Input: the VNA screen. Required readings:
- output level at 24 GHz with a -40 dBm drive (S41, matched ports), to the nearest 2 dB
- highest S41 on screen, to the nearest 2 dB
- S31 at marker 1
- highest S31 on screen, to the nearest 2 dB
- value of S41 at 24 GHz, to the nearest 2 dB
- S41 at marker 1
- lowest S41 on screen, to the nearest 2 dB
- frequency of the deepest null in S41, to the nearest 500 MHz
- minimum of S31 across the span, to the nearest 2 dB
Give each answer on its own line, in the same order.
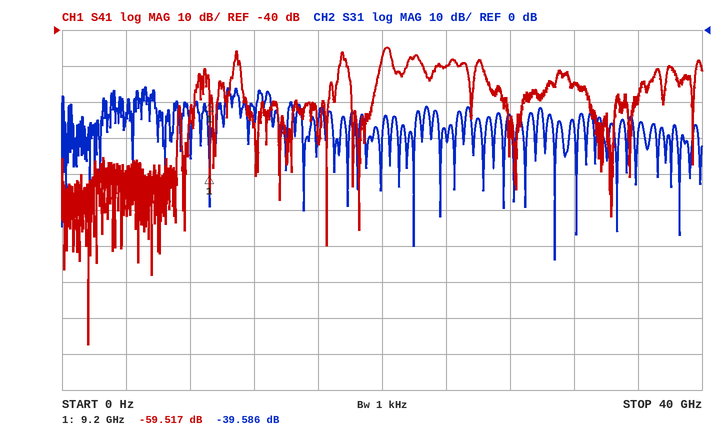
-90 dBm
-44 dB
-39.586 dB
-16 dB
-50 dB
-59.517 dB
-128 dB
1.5 GHz
-64 dB
